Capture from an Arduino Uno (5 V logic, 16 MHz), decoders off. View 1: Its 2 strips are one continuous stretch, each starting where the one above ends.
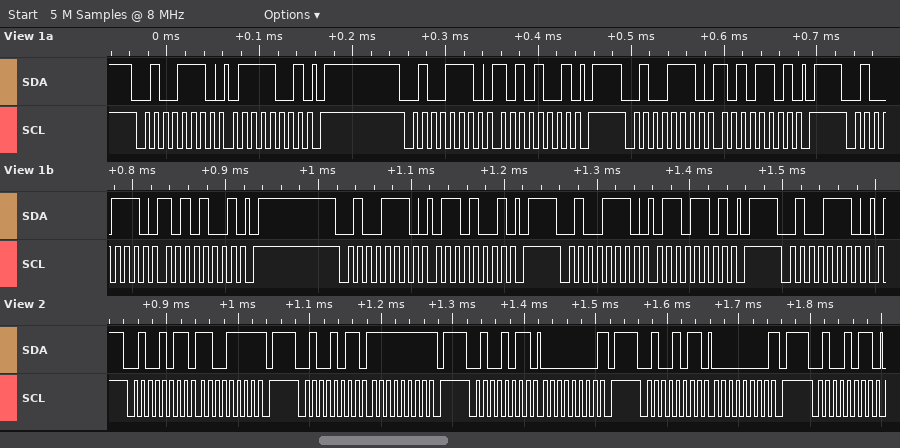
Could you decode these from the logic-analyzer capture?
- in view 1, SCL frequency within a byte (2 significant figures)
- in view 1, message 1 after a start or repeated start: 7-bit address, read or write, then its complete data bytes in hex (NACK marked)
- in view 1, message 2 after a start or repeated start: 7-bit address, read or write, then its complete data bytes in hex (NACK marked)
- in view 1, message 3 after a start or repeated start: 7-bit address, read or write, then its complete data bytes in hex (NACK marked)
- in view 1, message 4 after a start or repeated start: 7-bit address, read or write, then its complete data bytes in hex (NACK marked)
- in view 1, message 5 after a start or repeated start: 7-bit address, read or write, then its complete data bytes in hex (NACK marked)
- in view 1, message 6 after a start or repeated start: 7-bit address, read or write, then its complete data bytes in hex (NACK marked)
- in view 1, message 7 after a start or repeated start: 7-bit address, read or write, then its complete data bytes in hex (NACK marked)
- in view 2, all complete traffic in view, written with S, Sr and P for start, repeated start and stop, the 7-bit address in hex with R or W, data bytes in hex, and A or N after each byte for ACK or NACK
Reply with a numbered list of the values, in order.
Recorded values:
1. 100 kHz
2. 0x27 write: 79
3. 0x27 write: A9
4. 0x27 write: AD
5. 0x27 write: A9
6. 0x27 write: 69
7. 0x27 write: 6D
8. 0x27 write
9. S 25R A CF N P S 25R A FF N P S 25R A 00 N P S 25R A 00 N P S 25R A
